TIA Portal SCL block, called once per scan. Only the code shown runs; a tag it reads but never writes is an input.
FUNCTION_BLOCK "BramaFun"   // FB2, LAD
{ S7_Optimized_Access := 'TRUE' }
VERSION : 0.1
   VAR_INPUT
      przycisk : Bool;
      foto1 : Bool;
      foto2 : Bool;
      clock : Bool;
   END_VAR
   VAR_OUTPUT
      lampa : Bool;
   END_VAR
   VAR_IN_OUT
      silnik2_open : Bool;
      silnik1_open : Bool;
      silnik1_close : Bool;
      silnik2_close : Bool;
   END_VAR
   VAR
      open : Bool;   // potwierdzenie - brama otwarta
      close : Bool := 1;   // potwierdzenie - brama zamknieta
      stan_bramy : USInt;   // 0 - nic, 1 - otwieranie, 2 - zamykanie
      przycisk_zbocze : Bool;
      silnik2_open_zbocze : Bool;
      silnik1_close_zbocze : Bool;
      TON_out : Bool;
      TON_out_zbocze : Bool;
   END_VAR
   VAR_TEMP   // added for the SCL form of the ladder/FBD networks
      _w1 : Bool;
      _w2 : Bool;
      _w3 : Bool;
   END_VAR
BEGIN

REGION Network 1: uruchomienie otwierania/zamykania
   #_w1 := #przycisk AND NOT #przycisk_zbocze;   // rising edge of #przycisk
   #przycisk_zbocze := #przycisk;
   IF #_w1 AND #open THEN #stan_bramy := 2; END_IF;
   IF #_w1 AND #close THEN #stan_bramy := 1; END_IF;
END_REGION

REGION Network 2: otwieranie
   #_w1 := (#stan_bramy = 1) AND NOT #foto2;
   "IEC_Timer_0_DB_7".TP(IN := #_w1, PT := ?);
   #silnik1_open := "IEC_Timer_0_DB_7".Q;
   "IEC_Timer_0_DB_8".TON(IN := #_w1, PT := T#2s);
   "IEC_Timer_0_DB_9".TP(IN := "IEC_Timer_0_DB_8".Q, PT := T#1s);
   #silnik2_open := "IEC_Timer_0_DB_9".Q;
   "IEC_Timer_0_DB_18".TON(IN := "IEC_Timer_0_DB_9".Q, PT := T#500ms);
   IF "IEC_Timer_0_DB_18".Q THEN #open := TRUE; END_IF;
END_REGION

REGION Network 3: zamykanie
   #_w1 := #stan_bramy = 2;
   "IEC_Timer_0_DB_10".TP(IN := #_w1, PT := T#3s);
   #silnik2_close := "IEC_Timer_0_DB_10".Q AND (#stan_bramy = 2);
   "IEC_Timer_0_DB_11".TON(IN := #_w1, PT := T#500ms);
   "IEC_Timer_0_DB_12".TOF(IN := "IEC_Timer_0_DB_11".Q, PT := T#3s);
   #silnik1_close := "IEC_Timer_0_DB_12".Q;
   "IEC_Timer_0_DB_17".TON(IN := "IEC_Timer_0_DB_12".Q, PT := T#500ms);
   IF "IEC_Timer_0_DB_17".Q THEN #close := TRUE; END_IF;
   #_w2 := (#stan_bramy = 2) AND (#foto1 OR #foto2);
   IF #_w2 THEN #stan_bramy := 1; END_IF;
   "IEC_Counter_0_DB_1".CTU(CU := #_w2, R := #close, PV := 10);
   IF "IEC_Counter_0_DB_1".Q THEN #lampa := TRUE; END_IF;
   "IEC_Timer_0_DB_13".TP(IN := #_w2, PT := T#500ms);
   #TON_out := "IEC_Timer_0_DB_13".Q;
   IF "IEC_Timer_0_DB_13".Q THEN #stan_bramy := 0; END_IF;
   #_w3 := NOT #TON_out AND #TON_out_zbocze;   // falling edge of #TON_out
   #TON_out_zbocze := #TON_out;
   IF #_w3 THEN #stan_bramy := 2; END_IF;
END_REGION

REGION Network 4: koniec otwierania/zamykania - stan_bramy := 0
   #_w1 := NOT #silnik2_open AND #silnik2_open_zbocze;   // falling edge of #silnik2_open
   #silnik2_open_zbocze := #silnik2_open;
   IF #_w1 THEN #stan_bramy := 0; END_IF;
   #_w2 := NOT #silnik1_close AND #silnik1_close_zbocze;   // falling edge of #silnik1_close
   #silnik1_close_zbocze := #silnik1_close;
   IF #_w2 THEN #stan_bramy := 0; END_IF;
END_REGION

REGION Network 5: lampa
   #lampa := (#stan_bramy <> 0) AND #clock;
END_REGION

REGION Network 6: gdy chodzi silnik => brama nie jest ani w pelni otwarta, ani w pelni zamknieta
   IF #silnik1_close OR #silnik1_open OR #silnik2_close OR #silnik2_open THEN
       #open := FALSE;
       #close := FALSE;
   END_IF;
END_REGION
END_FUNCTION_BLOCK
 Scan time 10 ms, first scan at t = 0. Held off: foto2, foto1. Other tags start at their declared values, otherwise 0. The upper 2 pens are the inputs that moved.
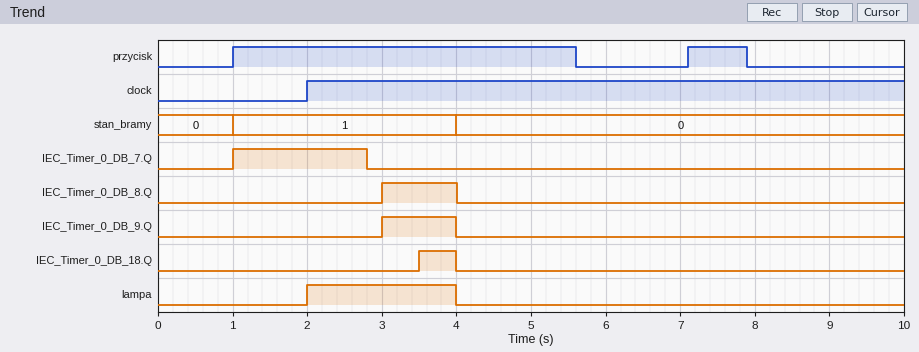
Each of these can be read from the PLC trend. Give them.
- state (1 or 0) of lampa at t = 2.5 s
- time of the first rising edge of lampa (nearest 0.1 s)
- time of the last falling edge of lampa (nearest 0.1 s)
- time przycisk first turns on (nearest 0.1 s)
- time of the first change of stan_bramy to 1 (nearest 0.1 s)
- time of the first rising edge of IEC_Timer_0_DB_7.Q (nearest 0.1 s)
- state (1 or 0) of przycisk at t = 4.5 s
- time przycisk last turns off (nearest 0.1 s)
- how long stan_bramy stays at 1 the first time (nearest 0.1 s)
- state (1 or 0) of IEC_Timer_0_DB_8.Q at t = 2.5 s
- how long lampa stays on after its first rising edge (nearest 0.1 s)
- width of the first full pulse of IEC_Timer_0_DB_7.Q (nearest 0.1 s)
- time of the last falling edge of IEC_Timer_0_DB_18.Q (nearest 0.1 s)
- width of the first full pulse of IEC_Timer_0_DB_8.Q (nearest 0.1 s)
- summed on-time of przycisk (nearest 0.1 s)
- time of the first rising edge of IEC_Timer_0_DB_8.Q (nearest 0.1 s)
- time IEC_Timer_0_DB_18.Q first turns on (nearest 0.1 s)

1
2.0 s
4.0 s
1.0 s
1.0 s
1.0 s
1
7.9 s
3.0 s
0
2.0 s
1.8 s
4.0 s
1.0 s
5.4 s
3.0 s
3.5 s
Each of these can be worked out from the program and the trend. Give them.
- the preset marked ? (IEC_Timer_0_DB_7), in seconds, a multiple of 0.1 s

1.8 s
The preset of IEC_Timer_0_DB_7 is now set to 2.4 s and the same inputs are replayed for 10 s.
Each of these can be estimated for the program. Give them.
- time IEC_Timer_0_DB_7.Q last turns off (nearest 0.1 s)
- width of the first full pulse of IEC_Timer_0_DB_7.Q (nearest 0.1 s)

3.4 s
2.4 s
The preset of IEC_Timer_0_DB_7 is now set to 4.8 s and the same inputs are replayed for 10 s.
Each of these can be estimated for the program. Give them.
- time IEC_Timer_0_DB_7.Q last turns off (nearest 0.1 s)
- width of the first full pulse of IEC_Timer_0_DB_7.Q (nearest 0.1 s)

5.8 s
4.8 s
